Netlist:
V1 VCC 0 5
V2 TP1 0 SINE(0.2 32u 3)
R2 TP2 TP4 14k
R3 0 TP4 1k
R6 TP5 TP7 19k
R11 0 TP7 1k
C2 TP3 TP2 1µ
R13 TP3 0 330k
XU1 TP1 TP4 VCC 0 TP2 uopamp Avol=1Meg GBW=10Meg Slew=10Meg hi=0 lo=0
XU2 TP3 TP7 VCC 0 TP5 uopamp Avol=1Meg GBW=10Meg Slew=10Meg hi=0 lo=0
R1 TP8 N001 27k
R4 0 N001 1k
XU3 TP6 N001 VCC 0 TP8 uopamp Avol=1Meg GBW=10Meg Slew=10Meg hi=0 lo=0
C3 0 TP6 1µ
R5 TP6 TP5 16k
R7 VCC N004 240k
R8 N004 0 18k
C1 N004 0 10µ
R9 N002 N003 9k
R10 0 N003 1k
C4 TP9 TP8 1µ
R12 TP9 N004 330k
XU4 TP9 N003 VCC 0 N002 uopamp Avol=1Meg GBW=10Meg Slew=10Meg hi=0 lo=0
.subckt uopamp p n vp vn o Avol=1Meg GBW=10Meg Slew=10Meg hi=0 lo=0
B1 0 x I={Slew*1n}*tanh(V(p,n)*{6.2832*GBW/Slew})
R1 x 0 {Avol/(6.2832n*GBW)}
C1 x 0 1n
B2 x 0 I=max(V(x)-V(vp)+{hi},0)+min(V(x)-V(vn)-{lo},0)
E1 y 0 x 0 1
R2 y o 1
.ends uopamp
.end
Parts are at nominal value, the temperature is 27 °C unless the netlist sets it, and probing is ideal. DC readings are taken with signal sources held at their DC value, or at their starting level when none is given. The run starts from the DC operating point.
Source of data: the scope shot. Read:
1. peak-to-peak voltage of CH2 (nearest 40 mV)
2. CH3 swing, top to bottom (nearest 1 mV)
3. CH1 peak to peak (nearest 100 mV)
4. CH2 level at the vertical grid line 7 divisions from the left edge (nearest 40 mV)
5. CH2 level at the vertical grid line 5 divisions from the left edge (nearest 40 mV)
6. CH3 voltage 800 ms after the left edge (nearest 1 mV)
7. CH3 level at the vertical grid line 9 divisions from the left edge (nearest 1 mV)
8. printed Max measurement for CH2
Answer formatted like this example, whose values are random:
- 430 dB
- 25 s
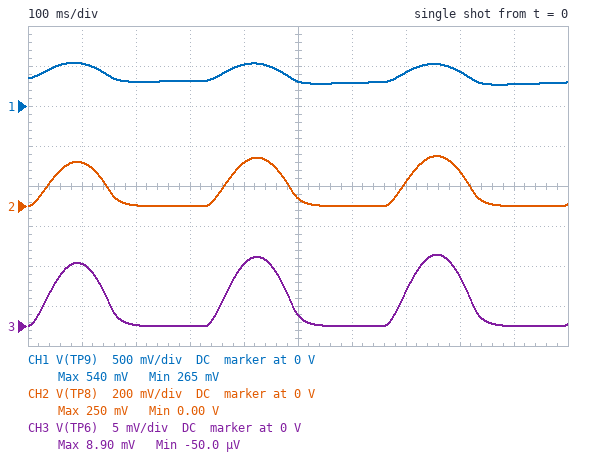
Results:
- 240 mV
- 9 mV
- 300 mV
- 120 mV
- 40 mV
- 6 mV
- 0 V
- 250 mV
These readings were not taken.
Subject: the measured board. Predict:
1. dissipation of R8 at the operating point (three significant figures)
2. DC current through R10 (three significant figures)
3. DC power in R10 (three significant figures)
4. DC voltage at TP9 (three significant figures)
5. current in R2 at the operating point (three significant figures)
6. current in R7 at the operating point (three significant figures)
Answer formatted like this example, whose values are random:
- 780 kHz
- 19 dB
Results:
- 6.76 µW
- 349 µA
- 122 µW
- 349 mV
- 200 µA
- 19.4 µA
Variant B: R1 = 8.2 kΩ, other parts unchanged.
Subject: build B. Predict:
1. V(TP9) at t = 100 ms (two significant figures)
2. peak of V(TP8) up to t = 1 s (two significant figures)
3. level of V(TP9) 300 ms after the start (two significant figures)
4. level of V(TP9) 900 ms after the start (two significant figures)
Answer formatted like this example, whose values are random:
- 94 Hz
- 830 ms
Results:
- 410 mV
- 82 mV
- 340 mV
- 320 mV
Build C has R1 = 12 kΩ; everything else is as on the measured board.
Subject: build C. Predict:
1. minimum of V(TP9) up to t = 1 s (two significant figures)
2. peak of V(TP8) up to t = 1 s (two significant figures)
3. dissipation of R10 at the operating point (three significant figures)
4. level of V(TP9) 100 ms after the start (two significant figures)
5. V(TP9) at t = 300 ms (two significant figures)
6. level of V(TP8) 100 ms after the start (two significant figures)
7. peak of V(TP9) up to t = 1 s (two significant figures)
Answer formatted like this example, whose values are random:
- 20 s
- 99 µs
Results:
- 310 mV
- 120 mV
- 122 µW
- 430 mV
- 330 mV
- 100 mV
- 440 mV
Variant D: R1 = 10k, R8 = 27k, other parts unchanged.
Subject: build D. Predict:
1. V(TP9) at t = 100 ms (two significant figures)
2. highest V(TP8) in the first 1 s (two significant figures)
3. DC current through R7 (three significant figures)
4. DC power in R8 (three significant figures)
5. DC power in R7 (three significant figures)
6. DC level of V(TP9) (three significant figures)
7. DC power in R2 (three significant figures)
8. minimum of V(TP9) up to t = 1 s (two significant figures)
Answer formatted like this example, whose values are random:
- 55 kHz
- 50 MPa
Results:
- 580 mV
- 98 mV
- 18.7 µA
- 9.47 µW
- 84.2 µW
- 506 mV
- 560 µW
- 470 mV
